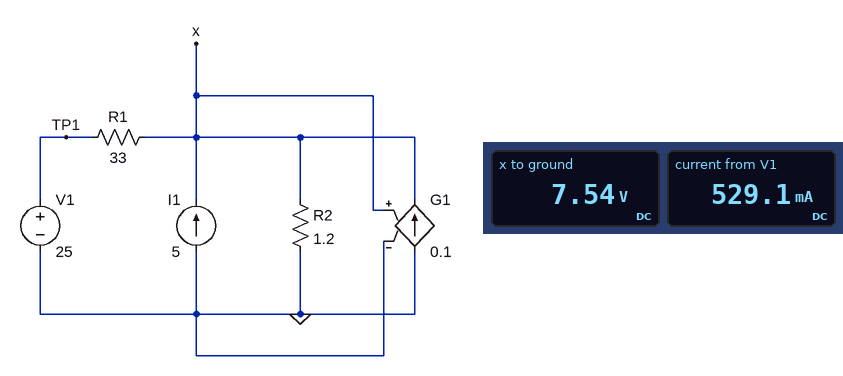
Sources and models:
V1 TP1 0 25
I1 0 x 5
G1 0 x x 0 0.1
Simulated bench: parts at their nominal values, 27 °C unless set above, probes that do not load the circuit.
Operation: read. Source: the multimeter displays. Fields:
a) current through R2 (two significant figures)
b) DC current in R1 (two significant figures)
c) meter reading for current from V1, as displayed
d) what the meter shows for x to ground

6.3 A
530 mA
529.1 mA
7.54 V
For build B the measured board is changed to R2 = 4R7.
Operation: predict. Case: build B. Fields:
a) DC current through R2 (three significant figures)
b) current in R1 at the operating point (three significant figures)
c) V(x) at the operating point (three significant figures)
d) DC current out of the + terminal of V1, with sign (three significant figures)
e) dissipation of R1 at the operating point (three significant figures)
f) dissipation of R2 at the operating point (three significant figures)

8.56 A
462 mA
40.2 V
-462 mA
7.04 W
345 W
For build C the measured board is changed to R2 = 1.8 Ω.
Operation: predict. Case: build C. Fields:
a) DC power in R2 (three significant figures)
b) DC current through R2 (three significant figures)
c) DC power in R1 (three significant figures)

78.0 W
6.58 A
5.24 W
